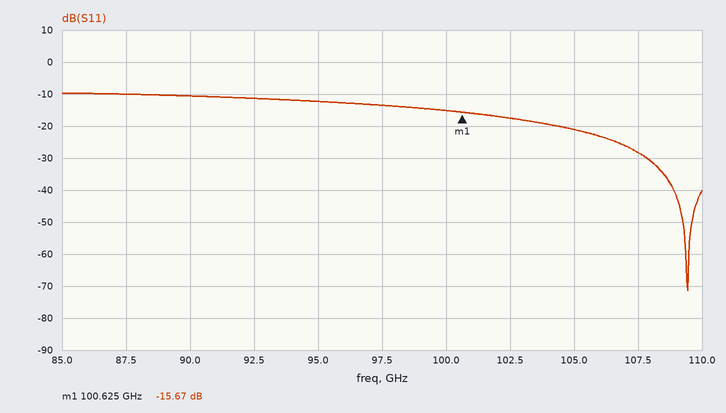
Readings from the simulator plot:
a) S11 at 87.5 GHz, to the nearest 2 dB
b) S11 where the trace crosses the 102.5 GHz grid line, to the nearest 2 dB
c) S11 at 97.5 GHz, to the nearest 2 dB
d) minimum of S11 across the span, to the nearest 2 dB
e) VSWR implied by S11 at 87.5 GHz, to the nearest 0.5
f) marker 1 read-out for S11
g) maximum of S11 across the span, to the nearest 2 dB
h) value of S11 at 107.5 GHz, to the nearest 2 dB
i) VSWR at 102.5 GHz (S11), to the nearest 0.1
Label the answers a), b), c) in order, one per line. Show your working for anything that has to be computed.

a) -10 dB
b) -18 dB
c) -14 dB
d) -72 dB
e) |Γ| = 10^(-10/20) = 0.3162; VSWR = (1 + 0.3162)/(1 − 0.3162) ≈ 1.92, so 2.0 to the nearest 0.5
f) -15.67 dB
g) -10 dB
h) -28 dB
i) |Γ| = 10^(-18/20) = 0.1259; VSWR = (1 + 0.1259)/(1 − 0.1259) ≈ 1.3
